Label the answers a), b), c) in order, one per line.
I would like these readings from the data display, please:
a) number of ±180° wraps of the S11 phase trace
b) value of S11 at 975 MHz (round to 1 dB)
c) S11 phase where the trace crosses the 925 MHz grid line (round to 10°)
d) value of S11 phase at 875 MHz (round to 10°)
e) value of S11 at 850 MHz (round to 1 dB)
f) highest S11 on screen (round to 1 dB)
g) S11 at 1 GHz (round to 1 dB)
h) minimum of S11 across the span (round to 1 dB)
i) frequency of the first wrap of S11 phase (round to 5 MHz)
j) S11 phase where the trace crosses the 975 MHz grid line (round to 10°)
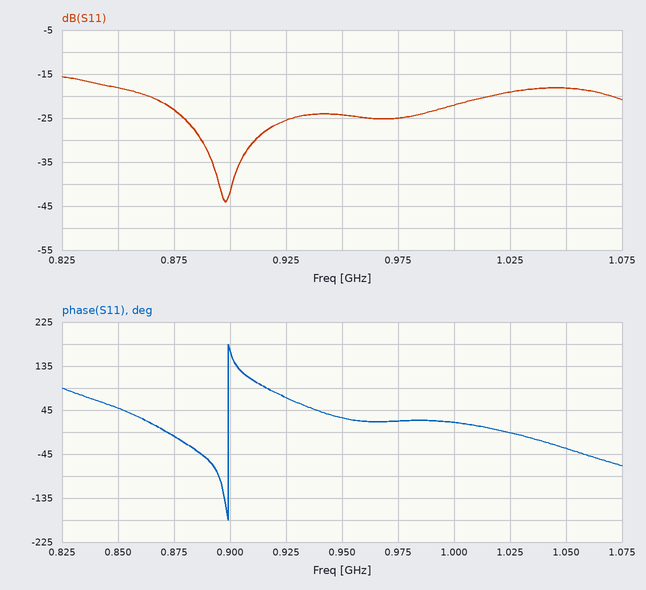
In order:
a) 1
b) -25 dB
c) 70°
d) -10°
e) -18 dB
f) -16 dB
g) -22 dB
h) -44 dB
i) 900 MHz
j) 20°
